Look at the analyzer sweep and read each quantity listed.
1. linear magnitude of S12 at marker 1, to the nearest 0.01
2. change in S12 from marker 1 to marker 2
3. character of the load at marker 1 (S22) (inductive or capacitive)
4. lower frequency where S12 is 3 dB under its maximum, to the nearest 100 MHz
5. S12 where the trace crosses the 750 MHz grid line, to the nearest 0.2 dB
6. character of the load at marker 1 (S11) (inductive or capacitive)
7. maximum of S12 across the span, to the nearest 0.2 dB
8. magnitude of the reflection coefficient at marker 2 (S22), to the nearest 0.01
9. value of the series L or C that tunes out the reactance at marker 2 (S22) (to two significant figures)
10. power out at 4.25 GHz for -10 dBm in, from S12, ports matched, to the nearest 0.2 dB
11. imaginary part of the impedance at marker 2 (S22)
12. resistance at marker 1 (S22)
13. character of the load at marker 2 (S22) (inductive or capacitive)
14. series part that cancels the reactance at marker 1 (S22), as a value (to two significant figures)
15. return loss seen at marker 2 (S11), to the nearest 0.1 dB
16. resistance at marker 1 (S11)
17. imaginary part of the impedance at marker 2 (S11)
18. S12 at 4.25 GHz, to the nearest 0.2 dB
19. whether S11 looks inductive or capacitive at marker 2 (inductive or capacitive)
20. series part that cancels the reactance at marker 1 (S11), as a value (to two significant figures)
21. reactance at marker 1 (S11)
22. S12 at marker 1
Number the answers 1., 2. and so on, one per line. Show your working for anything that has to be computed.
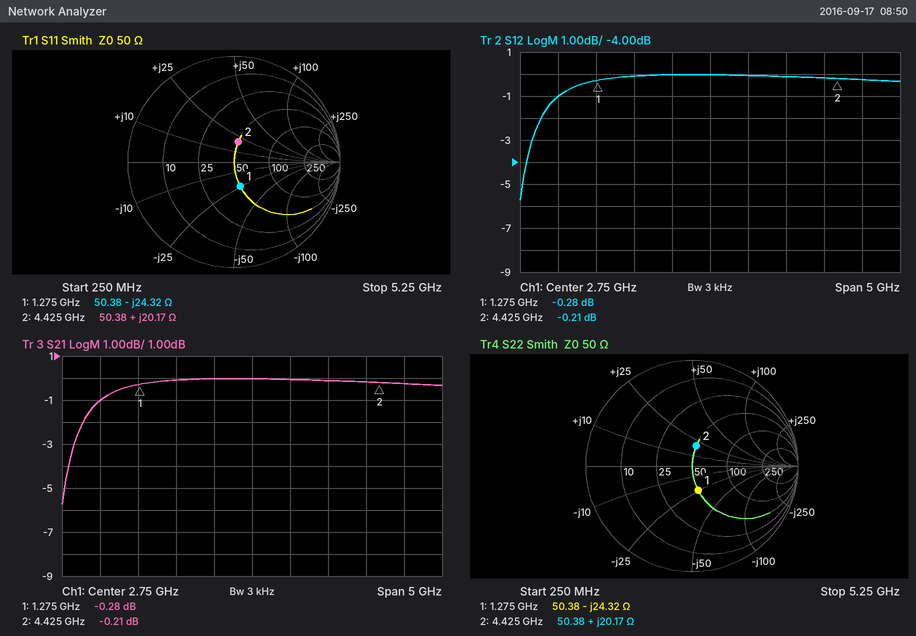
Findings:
1. 10^(-0.28/20) ≈ 0.97
2. -0.21 − (-0.28) = 0.07 dB
3. capacitive
4. 400 MHz
5. -1.0 dB
6. capacitive
7. 0.0 dB
8. 0.20
9. C = 1/(2π × 4.425 GHz × 20.17 Ω) ≈ 1.8 pF
10. -10 dBm + (-0.2 dB) = -10.2 dBm
11. +20.17 Ω
12. 50.38 Ω
13. inductive
14. L = 24.32 Ω/(2π × 1.275 GHz) ≈ 3.0 nH
15. 14.1 dB
16. 50.38 Ω
17. +20.17 Ω
18. -0.2 dB
19. inductive
20. L = 24.32 Ω/(2π × 1.275 GHz) ≈ 3.0 nH
21. -24.32 Ω
22. -0.28 dB
